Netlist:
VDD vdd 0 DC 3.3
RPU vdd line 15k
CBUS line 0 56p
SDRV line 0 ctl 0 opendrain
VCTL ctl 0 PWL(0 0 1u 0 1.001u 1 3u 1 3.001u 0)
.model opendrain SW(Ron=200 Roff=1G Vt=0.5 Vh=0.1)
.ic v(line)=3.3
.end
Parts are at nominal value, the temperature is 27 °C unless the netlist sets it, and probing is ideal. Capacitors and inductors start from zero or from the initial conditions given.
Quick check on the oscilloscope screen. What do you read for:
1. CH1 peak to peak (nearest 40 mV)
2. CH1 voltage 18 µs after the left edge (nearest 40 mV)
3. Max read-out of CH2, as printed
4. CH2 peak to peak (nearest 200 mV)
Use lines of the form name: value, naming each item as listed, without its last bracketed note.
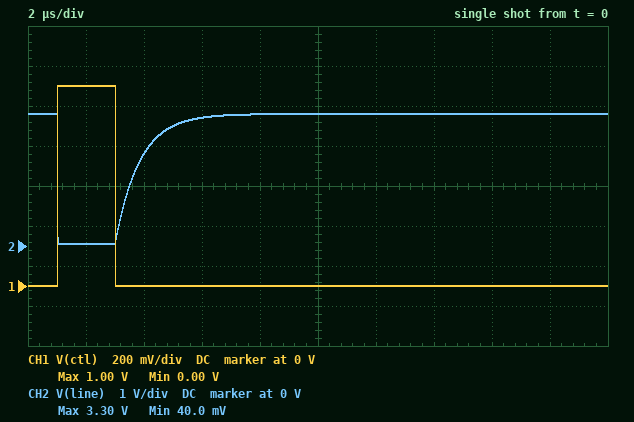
CH1 peak to peak: 1.00 V
CH1 voltage 18 µs after the left edge: 0 V
Max read-out of CH2, as printed: 3.30 V
CH2 peak to peak: 3.2 V
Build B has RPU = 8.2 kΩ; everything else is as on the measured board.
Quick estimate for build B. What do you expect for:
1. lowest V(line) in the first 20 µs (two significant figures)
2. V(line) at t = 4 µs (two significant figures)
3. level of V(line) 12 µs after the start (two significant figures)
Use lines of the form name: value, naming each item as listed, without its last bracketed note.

lowest V(line) in the first 20 µs: 79 mV
V(line) at t = 4 µs: 2.9 V
level of V(line) 12 µs after the start: 3.3 V
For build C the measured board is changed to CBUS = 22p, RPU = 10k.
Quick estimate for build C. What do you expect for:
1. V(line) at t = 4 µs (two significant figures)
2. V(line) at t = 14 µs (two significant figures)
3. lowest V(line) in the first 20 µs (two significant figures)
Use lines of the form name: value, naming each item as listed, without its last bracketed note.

V(line) at t = 4 µs: 3.3 V
V(line) at t = 14 µs: 3.3 V
lowest V(line) in the first 20 µs: 65 mV
